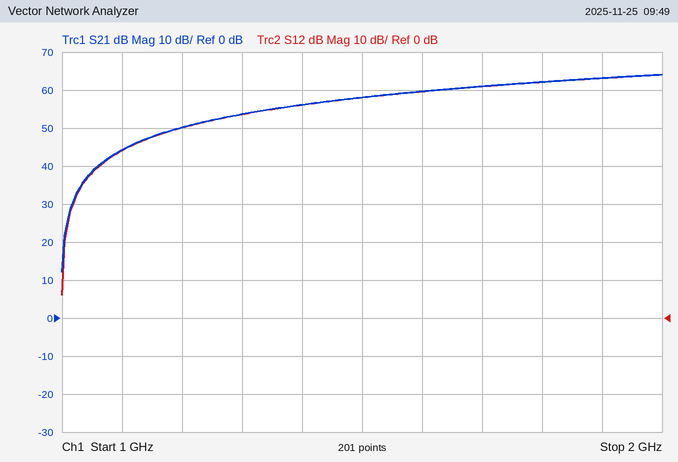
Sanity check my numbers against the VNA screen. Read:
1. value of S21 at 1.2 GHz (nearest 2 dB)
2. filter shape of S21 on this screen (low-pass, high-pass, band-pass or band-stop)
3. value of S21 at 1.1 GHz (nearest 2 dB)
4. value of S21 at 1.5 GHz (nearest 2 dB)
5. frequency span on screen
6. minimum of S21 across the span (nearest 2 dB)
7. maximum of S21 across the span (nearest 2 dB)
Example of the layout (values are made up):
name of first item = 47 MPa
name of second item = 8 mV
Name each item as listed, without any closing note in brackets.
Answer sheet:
value of S21 at 1.2 GHz = 50 dB
filter shape of S21 on this screen = high-pass
value of S21 at 1.1 GHz = 44 dB
value of S21 at 1.5 GHz = 58 dB
frequency span on screen = 1 GHz
minimum of S21 across the span = 12 dB
maximum of S21 across the span = 64 dB
